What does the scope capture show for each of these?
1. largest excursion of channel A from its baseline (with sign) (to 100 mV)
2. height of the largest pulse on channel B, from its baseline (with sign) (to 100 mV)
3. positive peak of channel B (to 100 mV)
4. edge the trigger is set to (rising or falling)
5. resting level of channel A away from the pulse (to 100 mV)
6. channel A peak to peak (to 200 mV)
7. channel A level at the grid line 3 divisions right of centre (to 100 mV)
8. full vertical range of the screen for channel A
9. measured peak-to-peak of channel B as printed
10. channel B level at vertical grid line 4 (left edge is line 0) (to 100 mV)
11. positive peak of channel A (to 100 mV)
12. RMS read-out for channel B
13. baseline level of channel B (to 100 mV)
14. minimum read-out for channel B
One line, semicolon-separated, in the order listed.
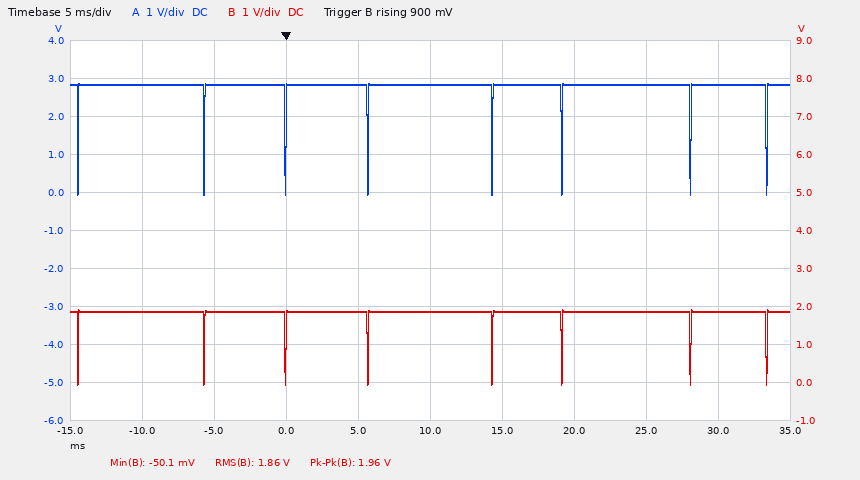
-2.9 V; -1.9 V; 1.9 V; rising; 2.8 V; 3.0 V; 2.8 V; 10 V; 1.96 V; 1.9 V; 2.9 V; 1.86 V; 1.9 V; -50.1 mV
